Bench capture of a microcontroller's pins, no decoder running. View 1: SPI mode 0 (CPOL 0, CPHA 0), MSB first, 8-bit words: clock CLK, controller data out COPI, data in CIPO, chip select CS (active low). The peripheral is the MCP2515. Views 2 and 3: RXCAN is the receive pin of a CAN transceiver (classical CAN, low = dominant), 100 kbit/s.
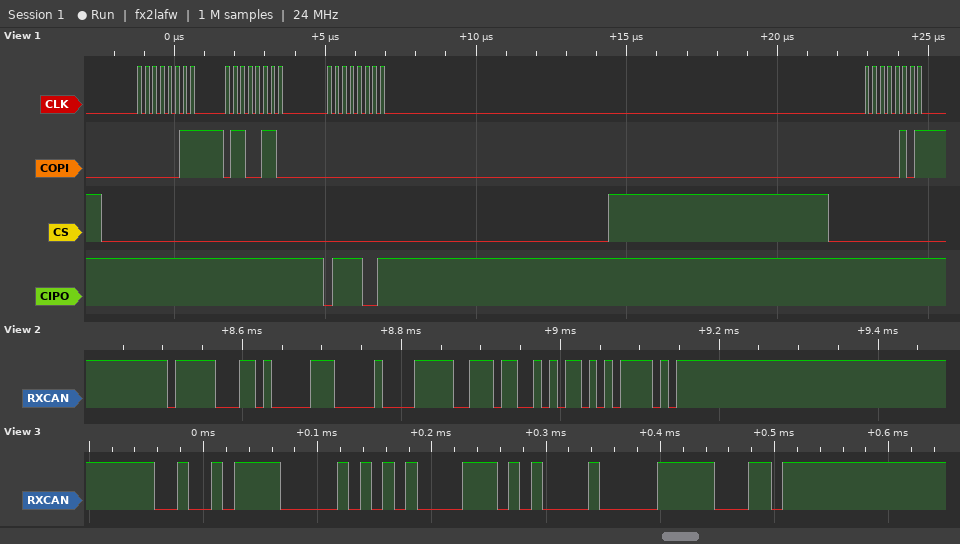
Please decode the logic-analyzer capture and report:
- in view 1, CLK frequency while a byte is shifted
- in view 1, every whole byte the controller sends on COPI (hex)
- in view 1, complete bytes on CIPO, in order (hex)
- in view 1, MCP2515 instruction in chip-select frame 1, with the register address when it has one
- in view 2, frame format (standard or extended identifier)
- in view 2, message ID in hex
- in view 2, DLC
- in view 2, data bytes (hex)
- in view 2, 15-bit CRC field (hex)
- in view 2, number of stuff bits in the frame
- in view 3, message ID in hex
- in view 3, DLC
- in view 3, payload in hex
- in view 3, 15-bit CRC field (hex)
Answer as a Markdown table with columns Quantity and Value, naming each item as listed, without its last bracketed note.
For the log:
| Quantity | Value |
|---|---|
| in view 1, CLK frequency while a byte is shifted | 4 MHz |
| in view 1, every whole byte the controller sends on COPI | 0x03 0x66 0x00 0x05 |
| in view 1, complete bytes on CIPO, in order | 0xFF 0xFF 0x79 0xFF |
| in view 1, MCP2515 instruction in chip-select frame 1, with the register address when it has one | READ 0x66 |
| in view 2, frame format | standard |
| in view 2, message ID in hex | 0x7CD |
| in view 2, DLC | 3 |
| in view 2, data bytes | 00 7D D9 |
| in view 2, 15-bit CRC field | 0x2D5E |
| in view 2, number of stuff bits in the frame | 4 |
| in view 3, message ID in hex | 0x25E |
| in view 3, DLC | 2 |
| in view 3, payload in hex | A1 D4 |
| in view 3, 15-bit CRC field | 0x1079 |
